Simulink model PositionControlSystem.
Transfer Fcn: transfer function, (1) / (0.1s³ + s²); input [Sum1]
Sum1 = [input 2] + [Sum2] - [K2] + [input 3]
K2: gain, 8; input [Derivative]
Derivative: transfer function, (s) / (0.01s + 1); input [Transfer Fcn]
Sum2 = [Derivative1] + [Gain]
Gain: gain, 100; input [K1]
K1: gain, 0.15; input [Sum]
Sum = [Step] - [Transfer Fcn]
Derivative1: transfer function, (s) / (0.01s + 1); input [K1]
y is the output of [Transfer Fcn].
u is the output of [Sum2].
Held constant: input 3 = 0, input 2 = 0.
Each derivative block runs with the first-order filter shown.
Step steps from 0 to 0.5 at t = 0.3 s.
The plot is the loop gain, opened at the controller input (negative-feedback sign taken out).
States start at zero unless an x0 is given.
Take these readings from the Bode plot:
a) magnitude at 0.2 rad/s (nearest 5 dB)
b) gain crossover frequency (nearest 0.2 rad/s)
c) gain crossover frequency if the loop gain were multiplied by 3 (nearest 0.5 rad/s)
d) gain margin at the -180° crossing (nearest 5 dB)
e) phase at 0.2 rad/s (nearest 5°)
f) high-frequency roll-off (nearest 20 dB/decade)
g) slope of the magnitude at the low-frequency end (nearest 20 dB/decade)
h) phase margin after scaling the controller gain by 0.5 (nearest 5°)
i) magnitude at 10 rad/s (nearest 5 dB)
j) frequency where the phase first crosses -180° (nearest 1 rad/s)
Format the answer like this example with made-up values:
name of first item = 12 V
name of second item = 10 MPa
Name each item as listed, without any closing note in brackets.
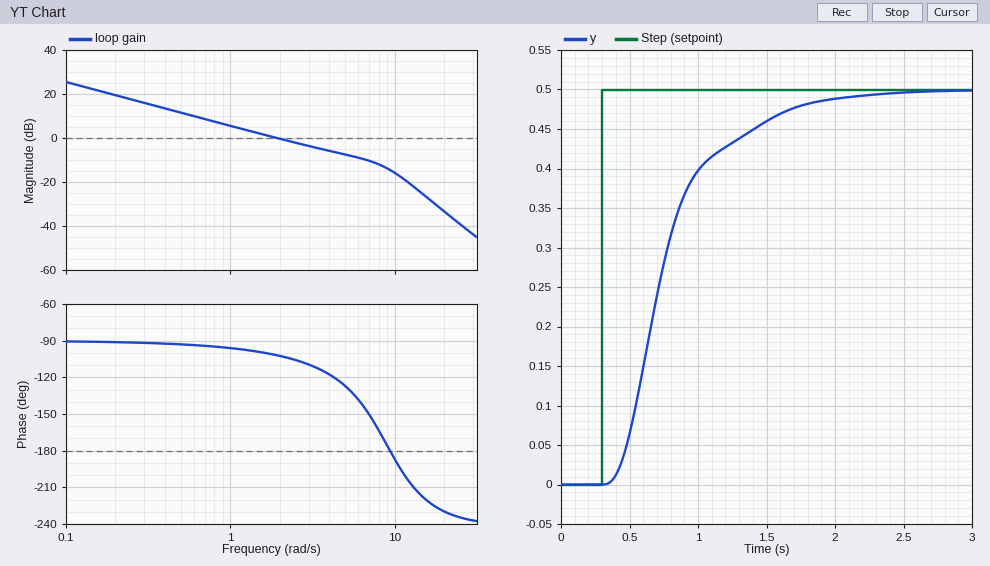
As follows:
magnitude at 0.2 rad/s = 20 dB
gain crossover frequency = 2.0 rad/s
gain crossover frequency if the loop gain were multiplied by 3 = 6.5 rad/s
gain margin at the -180° crossing = 15 dB
phase at 0.2 rad/s = -90°
high-frequency roll-off = -60 dB/decade
slope of the magnitude at the low-frequency end = -20 dB/decade
phase margin after scaling the controller gain by 0.5 = 85°
magnitude at 10 rad/s = -15 dB
frequency where the phase first crosses -180° = 9 rad/s
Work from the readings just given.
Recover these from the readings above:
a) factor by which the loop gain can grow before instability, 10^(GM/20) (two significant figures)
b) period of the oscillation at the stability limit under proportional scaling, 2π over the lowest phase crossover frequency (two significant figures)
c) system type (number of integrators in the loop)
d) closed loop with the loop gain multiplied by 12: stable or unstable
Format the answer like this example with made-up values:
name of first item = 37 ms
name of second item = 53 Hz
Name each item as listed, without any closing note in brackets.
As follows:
factor by which the loop gain can grow before instability, 10^(GM/20) = 5.6
period of the oscillation at the stability limit under proportional scaling, 2π over the lowest phase crossover frequency = 0.70 s
system type = 1
closed loop with the loop gain multiplied by 12: stable or unstable = unstable
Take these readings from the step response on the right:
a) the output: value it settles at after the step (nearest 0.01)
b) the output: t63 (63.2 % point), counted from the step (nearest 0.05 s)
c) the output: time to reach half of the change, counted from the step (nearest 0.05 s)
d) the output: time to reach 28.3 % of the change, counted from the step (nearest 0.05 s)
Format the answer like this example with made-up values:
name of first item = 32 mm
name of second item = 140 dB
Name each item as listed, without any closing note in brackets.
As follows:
the output: value it settles at after the step = 0.50
the output: t63 (63.2 % point), counted from the step = 0.50 s
the output: time to reach half of the change, counted from the step = 0.40 s
the output: time to reach 28.3 % of the change, counted from the step = 0.30 s
